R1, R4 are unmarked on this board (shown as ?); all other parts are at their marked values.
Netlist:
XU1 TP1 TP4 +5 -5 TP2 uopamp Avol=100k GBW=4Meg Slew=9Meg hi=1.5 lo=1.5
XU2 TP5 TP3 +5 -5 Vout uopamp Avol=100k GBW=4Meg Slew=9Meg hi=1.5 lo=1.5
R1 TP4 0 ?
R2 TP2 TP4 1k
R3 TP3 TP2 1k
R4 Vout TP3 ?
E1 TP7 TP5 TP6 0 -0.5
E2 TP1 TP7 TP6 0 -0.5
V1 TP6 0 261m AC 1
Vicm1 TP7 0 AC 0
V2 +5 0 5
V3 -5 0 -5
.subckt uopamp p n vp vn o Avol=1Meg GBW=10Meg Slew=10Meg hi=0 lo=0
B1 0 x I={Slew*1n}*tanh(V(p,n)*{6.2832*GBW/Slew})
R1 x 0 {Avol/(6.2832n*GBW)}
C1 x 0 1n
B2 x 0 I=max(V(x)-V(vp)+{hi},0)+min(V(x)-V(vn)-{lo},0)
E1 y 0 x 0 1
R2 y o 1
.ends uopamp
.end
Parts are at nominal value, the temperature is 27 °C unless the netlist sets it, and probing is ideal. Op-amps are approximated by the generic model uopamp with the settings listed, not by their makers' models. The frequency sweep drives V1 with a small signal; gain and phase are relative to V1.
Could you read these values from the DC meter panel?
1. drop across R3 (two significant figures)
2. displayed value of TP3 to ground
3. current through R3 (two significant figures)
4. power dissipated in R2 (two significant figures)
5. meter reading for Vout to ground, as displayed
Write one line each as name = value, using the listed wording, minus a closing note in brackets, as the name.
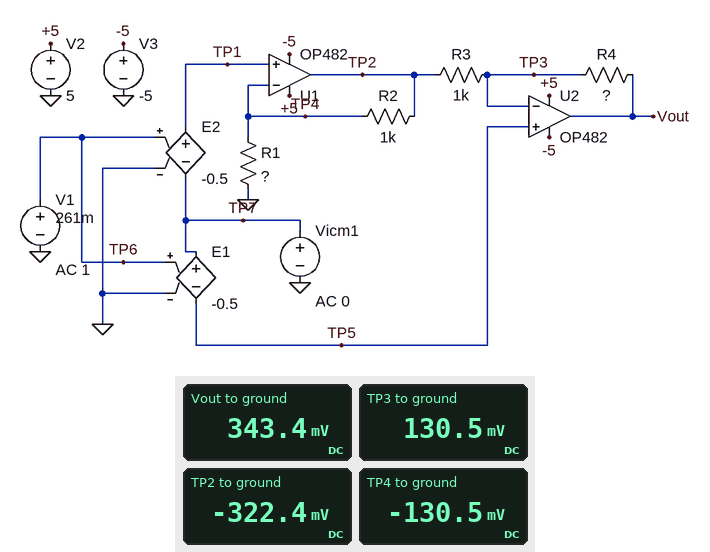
drop across R3 = 450 mV
displayed value of TP3 to ground = 130.5 mV
current through R3 = 450 µA
power dissipated in R2 = 37 µW
meter reading for Vout to ground, as displayed = 343.4 mV
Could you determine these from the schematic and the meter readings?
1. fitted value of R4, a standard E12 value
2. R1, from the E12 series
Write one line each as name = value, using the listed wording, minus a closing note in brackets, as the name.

fitted value of R4, a standard E12 value = 470 Ω
R1, from the E12 series = 680 Ω
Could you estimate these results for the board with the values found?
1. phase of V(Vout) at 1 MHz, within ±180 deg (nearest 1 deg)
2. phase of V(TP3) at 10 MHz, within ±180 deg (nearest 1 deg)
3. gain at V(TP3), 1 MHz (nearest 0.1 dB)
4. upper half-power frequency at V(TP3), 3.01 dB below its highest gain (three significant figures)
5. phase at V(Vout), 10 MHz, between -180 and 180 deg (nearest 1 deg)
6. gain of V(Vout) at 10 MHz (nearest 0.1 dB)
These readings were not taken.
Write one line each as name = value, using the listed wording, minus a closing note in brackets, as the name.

phase of V(Vout) at 1 MHz, within ±180 deg = -33 deg
phase of V(TP3) at 10 MHz, within ±180 deg = -83 deg
gain at V(TP3), 1 MHz = -7.5 dB
upper half-power frequency at V(TP3), 3.01 dB below its highest gain = 1.53 MHz
phase at V(Vout), 10 MHz, between -180 and 180 deg = -82 deg
gain of V(Vout) at 10 MHz = -14.1 dB
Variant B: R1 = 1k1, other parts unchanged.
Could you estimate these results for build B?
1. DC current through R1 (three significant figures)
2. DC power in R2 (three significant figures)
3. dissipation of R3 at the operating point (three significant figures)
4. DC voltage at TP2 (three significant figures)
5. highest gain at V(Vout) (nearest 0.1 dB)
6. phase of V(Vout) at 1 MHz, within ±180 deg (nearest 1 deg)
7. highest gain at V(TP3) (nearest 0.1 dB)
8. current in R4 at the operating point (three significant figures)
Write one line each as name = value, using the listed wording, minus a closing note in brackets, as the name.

DC current through R1 = 119 µA
DC power in R2 = 14.1 µW
dissipation of R3 at the operating point = 144 µW
DC voltage at TP2 = -249 mV
highest gain at V(Vout) = 1.5 dB
phase of V(Vout) at 1 MHz, within ±180 deg = -29 deg
highest gain at V(TP3) = -6.0 dB
current in R4 at the operating point = 380 µA
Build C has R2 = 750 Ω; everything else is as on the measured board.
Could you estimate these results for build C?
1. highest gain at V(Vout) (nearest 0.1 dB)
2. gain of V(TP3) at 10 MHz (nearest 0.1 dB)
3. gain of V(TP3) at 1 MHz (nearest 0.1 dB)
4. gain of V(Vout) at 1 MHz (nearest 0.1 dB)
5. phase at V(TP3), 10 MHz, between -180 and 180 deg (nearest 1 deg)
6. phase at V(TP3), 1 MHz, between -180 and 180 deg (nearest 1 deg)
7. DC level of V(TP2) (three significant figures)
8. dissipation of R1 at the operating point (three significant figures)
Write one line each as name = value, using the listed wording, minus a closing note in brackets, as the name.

highest gain at V(Vout) = 1.8 dB
gain of V(TP3) at 10 MHz = -22.8 dB
gain of V(TP3) at 1 MHz = -7.3 dB
gain of V(Vout) at 1 MHz = 0.6 dB
phase at V(TP3), 10 MHz, between -180 and 180 deg = -84 deg
phase at V(TP3), 1 MHz, between -180 and 180 deg = -32 deg
DC level of V(TP2) = -274 mV
dissipation of R1 at the operating point = 25.0 µW
